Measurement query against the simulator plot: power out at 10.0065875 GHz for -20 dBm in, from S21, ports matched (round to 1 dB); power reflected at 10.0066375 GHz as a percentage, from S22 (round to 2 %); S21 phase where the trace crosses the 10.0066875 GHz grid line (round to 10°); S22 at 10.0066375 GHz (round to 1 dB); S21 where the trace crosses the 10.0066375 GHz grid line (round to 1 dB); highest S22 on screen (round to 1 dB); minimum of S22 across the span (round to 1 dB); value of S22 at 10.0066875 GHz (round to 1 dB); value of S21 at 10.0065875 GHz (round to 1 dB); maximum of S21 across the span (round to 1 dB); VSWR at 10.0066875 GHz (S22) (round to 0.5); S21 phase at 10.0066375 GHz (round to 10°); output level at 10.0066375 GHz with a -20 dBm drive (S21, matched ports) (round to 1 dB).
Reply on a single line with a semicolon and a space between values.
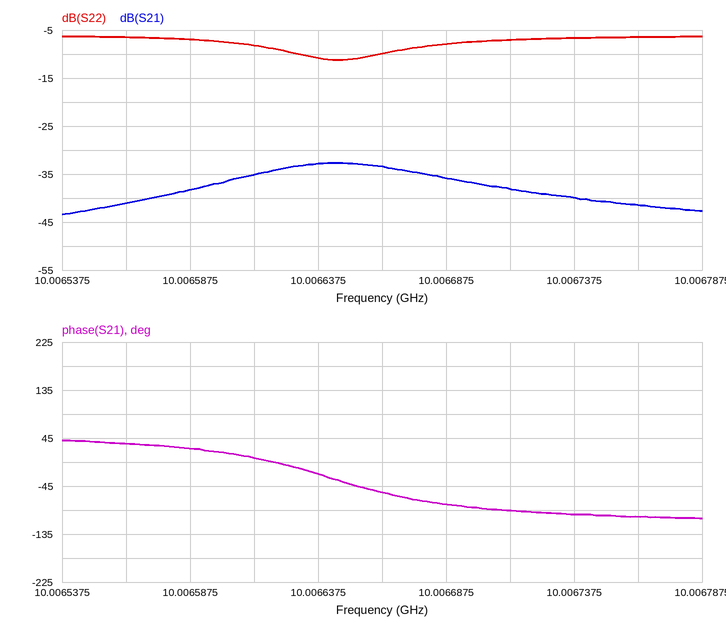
-58 dBm; 8 %; -80°; -11 dB; -33 dB; -6 dB; -11 dB; -8 dB; -38 dB; -33 dB; 2.5; -20°; -53 dBm
